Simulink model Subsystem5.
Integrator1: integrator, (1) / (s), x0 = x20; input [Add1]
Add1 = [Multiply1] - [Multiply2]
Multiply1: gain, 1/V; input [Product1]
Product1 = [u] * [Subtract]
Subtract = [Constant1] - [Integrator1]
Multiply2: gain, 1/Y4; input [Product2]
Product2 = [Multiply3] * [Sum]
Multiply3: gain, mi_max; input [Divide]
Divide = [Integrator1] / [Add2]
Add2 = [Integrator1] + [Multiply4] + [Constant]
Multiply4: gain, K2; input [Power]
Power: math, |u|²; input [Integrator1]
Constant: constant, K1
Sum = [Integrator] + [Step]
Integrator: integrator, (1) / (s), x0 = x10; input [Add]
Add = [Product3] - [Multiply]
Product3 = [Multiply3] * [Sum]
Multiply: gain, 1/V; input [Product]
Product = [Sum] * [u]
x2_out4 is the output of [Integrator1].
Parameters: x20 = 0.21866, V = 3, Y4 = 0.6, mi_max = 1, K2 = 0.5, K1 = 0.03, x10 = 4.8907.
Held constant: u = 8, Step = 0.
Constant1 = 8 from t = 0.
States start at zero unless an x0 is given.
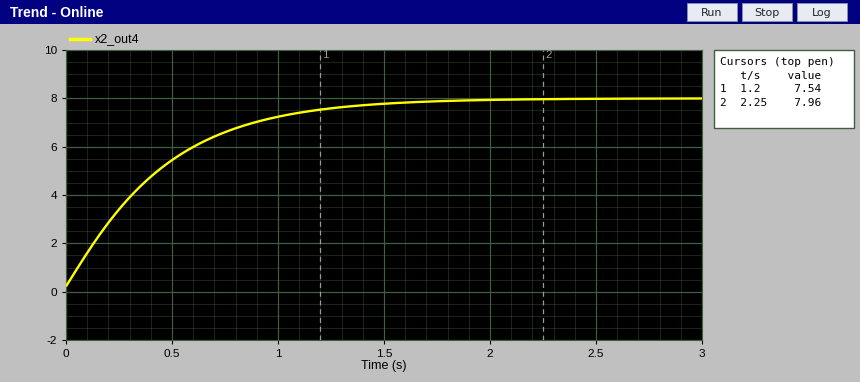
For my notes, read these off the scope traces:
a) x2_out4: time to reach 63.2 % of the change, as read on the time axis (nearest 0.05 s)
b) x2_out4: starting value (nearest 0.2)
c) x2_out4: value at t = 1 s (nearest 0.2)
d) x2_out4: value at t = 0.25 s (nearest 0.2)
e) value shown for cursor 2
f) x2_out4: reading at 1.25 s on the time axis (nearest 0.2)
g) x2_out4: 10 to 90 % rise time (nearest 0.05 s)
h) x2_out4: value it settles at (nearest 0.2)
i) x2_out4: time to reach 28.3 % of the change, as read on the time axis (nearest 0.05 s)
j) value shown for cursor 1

0.45 s
0.2
7.2
3.4
7.96
7.6
0.95 s
8.0
0.15 s
7.54
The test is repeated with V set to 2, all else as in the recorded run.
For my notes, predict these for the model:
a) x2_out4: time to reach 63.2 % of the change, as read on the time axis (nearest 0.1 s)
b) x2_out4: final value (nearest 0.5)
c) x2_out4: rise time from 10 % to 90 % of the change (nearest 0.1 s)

0.3 s
8.0
0.6 s
